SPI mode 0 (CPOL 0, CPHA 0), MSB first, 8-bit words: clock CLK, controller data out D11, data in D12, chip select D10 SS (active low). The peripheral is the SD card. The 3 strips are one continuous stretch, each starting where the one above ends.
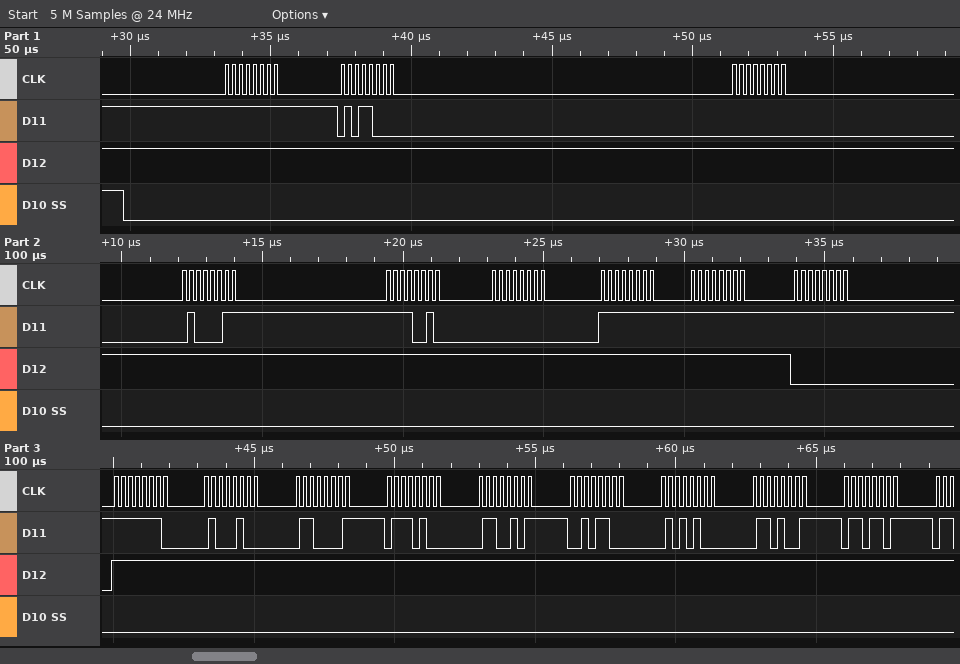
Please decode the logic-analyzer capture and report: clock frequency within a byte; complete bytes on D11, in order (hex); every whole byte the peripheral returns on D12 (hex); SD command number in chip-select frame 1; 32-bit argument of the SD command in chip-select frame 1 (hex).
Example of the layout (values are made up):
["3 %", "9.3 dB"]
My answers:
["4 MHz", "0xFF 0x58 0x00 0x43 0xF2 0x00 0xFF 0xFF 0xFF 0xFE 0x44 0x61 0x74 0x65 0x2C 0x54 0x69 0x6D", "0xFF 0xFF 0xFF 0xFF 0xFF 0xFF 0xFF 0xFF 0x00 0xFF 0xFF 0xFF 0xFF 0xFF 0xFF 0xFF 0xFF 0xFF", "CMD24", "0x0043F200"]
